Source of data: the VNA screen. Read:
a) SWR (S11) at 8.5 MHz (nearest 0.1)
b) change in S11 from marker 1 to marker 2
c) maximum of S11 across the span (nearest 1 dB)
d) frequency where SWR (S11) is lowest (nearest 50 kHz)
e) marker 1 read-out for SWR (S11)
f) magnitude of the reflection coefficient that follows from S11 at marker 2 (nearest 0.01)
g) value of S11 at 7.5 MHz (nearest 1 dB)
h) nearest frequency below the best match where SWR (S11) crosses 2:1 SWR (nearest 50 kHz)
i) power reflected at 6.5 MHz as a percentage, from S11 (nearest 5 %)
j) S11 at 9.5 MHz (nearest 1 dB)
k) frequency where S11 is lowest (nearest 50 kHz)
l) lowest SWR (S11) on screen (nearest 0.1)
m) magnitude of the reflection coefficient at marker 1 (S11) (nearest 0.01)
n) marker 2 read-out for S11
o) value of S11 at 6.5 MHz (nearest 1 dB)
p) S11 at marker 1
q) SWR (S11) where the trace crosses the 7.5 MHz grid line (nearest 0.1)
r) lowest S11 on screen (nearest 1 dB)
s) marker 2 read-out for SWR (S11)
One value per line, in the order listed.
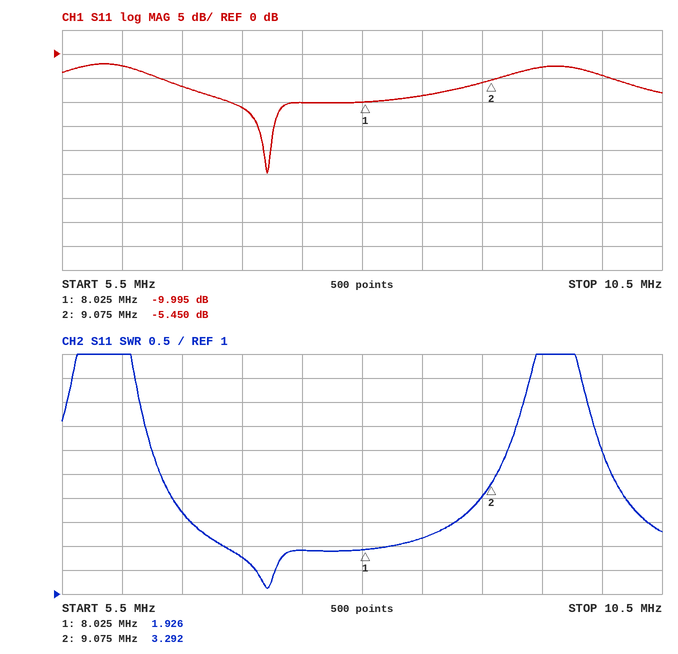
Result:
2.2
4.545 dB
-2 dB
7.20 MHz
1.926
0.53
-10 dB
6.85 MHz
20 %
-3 dB
7.20 MHz
1.1
0.32
-5.450 dB
-7 dB
-9.995 dB
1.9
-25 dB
3.292
